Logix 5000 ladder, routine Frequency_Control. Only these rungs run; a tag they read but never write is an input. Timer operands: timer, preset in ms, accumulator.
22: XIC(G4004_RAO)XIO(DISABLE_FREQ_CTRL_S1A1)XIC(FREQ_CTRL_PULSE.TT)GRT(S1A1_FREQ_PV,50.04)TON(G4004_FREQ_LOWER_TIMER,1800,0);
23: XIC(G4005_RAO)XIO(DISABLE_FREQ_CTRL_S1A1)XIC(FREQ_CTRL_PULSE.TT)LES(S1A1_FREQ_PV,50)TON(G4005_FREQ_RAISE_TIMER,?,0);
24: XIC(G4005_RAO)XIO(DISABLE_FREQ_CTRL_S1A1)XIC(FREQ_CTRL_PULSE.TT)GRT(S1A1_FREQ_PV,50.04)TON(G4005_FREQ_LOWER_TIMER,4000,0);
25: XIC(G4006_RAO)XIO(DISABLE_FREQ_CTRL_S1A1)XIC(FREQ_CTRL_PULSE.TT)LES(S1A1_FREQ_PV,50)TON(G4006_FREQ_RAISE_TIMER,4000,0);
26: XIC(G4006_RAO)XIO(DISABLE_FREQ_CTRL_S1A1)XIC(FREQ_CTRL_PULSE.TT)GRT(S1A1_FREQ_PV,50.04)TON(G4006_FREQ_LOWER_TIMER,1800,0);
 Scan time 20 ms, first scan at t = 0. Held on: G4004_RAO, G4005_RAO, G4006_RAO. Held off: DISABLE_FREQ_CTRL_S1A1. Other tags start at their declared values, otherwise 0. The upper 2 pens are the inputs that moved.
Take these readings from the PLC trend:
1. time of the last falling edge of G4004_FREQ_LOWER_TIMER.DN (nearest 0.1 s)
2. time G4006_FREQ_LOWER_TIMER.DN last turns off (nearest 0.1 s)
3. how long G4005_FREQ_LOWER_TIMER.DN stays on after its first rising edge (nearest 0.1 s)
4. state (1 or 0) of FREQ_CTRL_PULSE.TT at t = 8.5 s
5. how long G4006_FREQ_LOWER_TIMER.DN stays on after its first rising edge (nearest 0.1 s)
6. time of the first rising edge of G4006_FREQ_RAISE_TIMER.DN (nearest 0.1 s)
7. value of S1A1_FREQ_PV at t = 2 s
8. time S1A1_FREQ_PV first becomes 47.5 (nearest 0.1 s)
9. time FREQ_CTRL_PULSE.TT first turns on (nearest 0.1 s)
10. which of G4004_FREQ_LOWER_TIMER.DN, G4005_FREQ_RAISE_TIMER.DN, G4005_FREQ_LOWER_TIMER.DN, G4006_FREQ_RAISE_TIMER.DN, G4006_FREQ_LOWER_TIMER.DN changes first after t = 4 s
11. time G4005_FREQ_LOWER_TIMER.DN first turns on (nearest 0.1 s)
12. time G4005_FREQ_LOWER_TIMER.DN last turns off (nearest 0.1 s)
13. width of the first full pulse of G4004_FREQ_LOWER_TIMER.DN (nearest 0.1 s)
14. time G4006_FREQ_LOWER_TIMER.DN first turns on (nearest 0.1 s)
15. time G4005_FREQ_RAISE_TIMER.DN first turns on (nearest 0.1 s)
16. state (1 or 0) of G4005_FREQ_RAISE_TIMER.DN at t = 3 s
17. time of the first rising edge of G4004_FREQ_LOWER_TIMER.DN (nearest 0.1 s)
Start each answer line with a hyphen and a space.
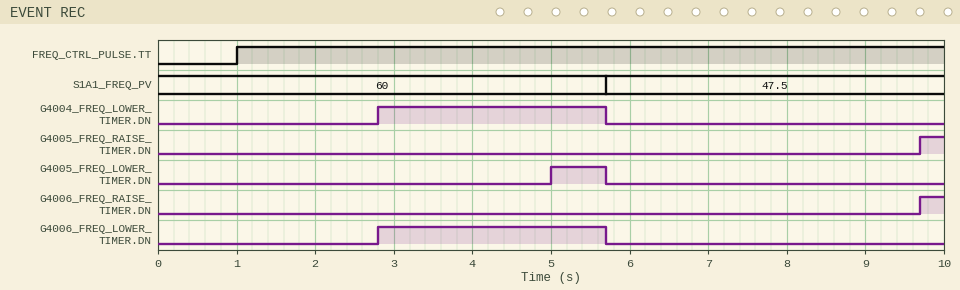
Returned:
- 5.7 s
- 5.7 s
- 0.7 s
- 1
- 2.9 s
- 9.7 s
- 60
- 5.7 s
- 1.0 s
- G4005_FREQ_LOWER_TIMER.DN
- 5.0 s
- 5.7 s
- 2.9 s
- 2.8 s
- 9.7 s
- 0
- 2.8 s
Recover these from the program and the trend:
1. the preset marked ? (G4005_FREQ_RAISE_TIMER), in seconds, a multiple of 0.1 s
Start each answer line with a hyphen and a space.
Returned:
- 4.0 s
